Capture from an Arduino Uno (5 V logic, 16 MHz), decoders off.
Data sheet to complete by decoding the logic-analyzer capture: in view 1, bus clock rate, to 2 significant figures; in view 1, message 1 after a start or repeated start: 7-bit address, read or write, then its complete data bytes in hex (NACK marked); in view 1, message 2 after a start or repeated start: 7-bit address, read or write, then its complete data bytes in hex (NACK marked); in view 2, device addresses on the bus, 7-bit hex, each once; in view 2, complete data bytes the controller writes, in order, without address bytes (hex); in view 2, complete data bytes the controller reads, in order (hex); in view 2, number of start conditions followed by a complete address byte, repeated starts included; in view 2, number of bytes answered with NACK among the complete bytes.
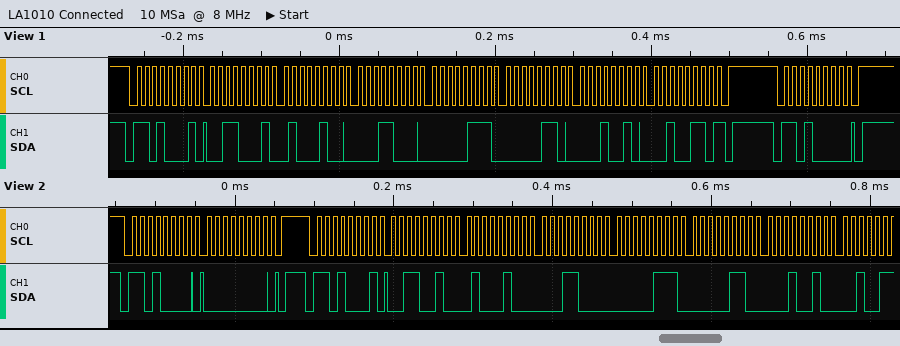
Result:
100 kHz
0x68 read: 31 44 18 07 06 12 26 NACK
0x68 write
0x68
00
32 44 18 07 06 12
2
0
